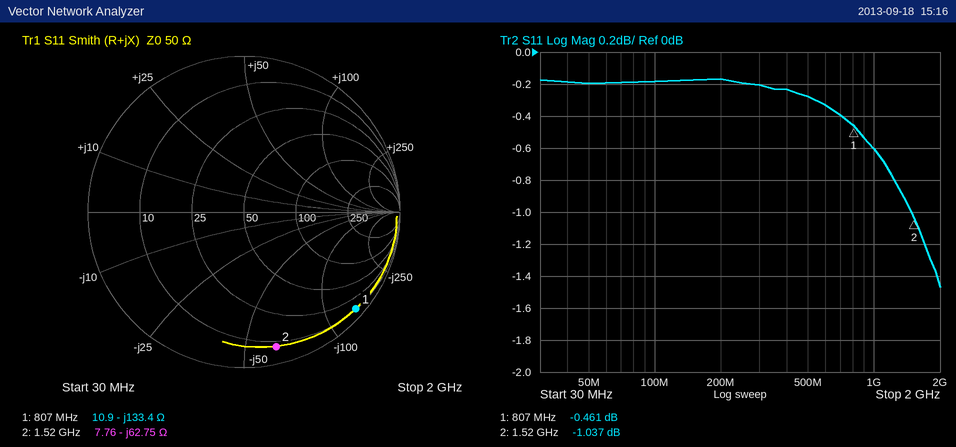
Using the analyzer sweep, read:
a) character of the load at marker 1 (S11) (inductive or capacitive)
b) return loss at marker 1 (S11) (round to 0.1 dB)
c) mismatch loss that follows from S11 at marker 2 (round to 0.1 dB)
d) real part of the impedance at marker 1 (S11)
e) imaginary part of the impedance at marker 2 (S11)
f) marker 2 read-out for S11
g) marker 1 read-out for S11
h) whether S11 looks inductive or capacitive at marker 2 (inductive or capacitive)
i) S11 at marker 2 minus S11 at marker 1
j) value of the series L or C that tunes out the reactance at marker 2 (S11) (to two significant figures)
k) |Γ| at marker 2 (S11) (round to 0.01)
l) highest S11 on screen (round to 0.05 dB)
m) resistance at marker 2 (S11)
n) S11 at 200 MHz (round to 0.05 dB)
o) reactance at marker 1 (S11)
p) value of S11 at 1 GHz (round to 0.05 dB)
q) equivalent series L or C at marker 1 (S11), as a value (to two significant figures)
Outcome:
capacitive
0.5 dB
6.7 dB
10.9 Ω
-62.75 Ω
-1.037 dB
-0.461 dB
capacitive
-0.576 dB
6.6 nH
0.89
-0.15 dB
7.76 Ω
-0.15 dB
-133.4 Ω
-0.60 dB
1.5 pF
